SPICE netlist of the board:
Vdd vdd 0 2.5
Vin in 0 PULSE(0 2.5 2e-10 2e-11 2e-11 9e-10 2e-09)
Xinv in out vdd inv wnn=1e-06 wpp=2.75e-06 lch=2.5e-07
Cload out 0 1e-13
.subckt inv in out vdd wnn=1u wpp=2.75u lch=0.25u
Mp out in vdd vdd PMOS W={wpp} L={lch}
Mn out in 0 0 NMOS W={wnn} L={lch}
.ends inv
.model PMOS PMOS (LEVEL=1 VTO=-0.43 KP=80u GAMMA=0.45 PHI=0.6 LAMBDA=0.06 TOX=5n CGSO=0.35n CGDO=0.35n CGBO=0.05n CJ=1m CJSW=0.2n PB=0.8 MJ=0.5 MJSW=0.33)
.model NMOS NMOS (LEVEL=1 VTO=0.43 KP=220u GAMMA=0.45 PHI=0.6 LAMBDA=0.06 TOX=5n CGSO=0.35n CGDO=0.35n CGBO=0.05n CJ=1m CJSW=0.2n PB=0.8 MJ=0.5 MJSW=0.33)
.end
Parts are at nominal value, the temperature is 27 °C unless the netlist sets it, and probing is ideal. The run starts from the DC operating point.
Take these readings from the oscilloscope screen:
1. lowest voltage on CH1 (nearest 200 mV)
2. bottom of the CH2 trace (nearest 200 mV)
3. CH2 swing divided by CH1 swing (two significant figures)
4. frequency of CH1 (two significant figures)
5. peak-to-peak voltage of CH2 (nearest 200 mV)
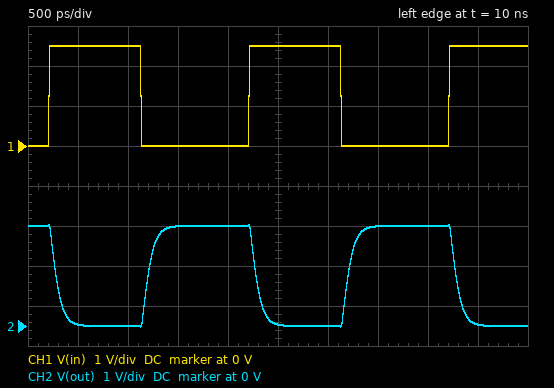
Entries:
0 V
0 V
1.0
500 MHz
2.6 V
